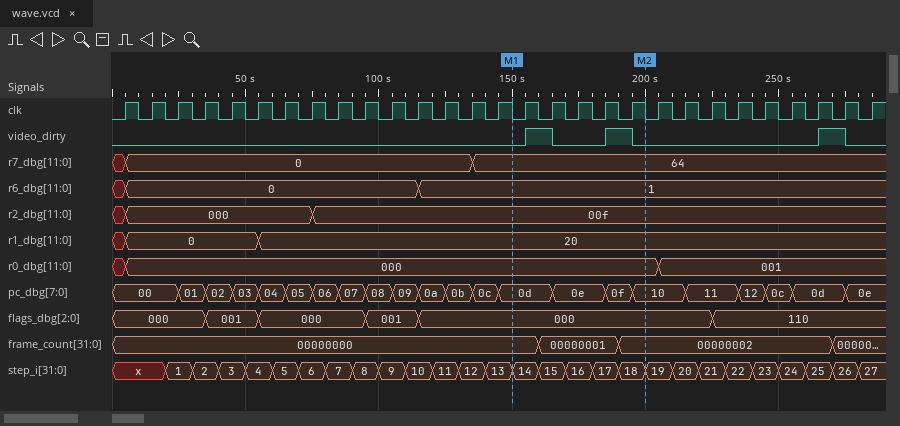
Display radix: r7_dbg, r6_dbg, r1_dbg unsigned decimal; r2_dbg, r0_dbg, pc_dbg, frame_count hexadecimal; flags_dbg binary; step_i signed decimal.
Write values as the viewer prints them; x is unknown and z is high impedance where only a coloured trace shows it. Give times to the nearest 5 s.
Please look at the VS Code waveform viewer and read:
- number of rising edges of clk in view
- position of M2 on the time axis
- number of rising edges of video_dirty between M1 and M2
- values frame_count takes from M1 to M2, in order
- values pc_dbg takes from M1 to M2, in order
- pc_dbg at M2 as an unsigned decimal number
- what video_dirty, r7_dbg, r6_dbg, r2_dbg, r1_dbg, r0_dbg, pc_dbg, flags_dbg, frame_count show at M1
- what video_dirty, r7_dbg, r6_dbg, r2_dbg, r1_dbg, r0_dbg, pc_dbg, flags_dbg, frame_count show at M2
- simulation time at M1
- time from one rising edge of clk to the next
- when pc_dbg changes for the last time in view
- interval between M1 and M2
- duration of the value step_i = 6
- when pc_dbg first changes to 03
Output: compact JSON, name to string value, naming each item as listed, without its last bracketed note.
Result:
{"number of rising edges of clk in view": "29", "position of M2 on the time axis": "200 s", "number of rising edges of video_dirty between M1 and M2": "2", "values frame_count takes from M1 to M2, in order": "00000000, 00000001, 00000002", "values pc_dbg takes from M1 to M2, in order": "0d, 0e, 0f, 10", "pc_dbg at M2 as an unsigned decimal number": "16", "what video_dirty, r7_dbg, r6_dbg, r2_dbg, r1_dbg, r0_dbg, pc_dbg, flags_dbg, frame_count show at M1": "video_dirty=0, r7_dbg=64, r6_dbg=1, r2_dbg=00f, r1_dbg=20, r0_dbg=000, pc_dbg=0d, flags_dbg=000, frame_count=00000000", "what video_dirty, r7_dbg, r6_dbg, r2_dbg, r1_dbg, r0_dbg, pc_dbg, flags_dbg, frame_count show at M2": "video_dirty=0, r7_dbg=64, r6_dbg=1, r2_dbg=00f, r1_dbg=20, r0_dbg=000, pc_dbg=10, flags_dbg=000, frame_count=00000002", "simulation time at M1": "150 s", "time from one rising edge of clk to the next": "10 s", "when pc_dbg changes for the last time in view": "275 s", "interval between M1 and M2": "50 s", "duration of the value step_i = 6": "10 s", "when pc_dbg first changes to 03": "45 s"}
